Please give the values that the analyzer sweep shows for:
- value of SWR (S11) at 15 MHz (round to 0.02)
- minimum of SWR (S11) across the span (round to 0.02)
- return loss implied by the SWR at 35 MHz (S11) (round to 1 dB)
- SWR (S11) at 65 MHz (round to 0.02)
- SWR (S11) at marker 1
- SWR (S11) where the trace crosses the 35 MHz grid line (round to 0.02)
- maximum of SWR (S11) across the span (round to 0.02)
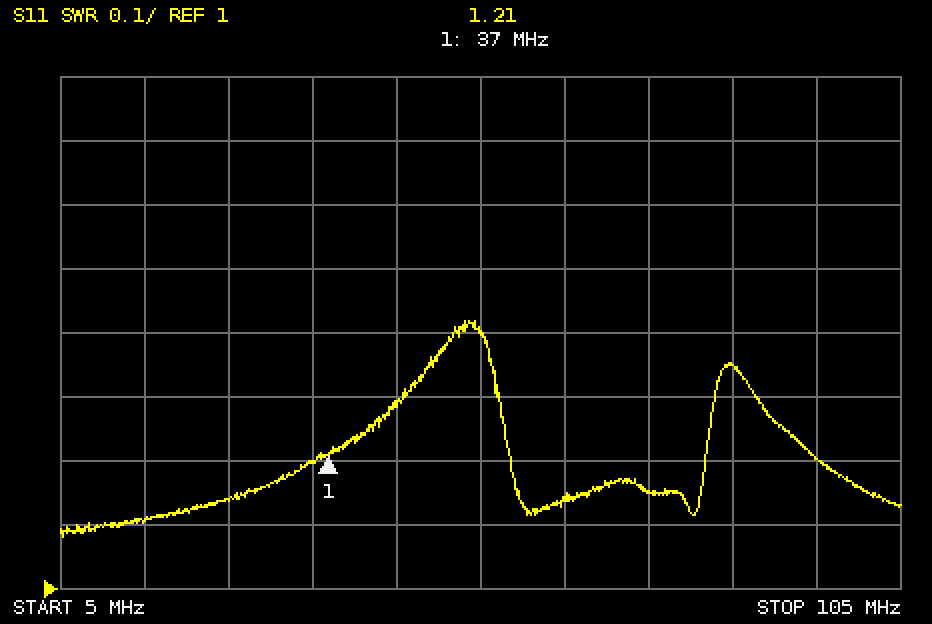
1.10
1.08
21 dB
1.14
1.21
1.20
1.42
